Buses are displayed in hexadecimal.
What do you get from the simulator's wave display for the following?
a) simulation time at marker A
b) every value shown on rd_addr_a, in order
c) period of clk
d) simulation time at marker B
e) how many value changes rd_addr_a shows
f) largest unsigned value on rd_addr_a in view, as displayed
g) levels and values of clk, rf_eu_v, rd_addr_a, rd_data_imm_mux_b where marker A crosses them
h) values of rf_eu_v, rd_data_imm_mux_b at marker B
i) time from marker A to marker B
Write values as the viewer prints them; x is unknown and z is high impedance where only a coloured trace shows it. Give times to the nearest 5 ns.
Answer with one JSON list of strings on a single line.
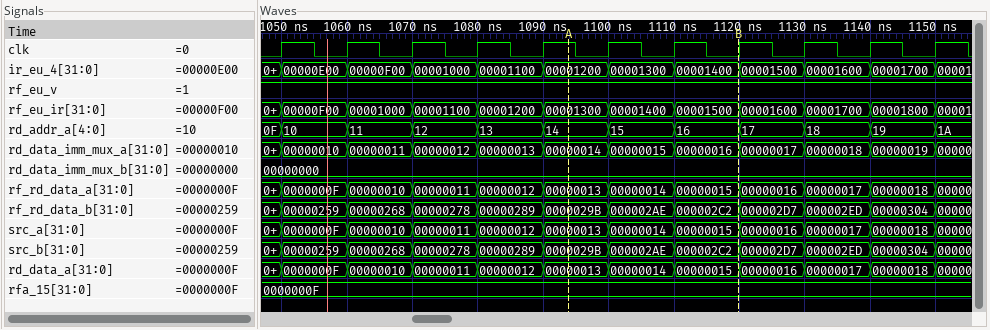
["1095 ns", "0F, 10, 11, 12, 13, 14, 15, 16, 17, 18, 19, 1A", "10 ns", "1120 ns", "11", "1A", "clk=1, rf_eu_v=1, rd_addr_a=14, rd_data_imm_mux_b=00000000", "rf_eu_v=1, rd_data_imm_mux_b=00000000", "25 ns"]
